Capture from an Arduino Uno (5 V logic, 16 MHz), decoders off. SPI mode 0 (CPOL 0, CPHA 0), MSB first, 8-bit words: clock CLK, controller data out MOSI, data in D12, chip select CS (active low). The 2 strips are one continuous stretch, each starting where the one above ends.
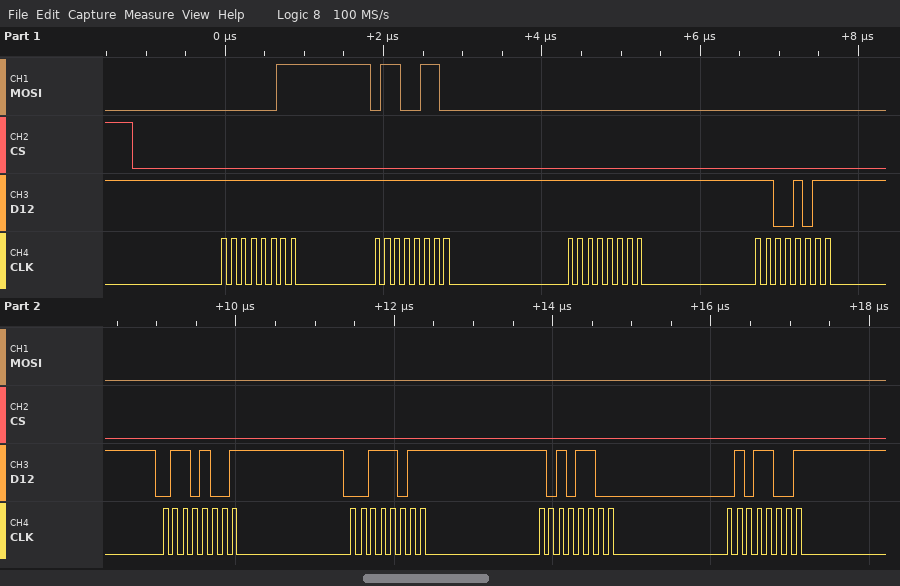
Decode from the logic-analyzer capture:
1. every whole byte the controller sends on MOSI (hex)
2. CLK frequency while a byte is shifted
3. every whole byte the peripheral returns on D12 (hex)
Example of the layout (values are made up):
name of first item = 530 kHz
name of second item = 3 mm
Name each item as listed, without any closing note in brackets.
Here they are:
every whole byte the controller sends on MOSI = 03 66 00 00 00 00 00 00
CLK frequency while a byte is shifted = 8 MHz
every whole byte the peripheral returns on D12 = FF FF FF CB 69 3B AC 59
